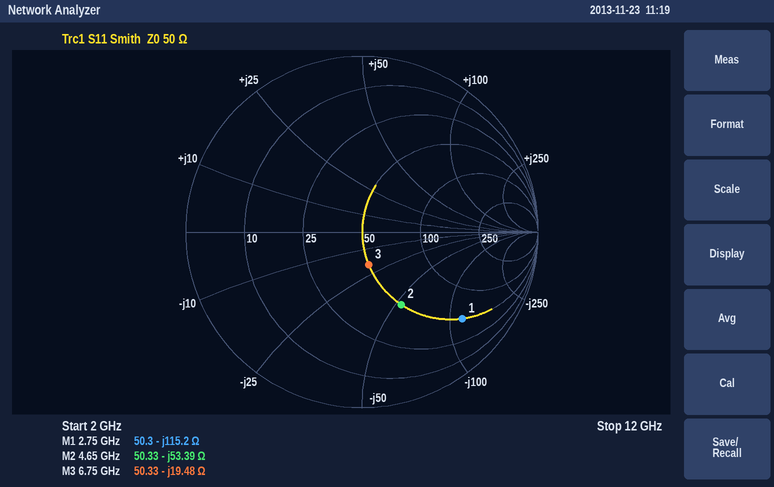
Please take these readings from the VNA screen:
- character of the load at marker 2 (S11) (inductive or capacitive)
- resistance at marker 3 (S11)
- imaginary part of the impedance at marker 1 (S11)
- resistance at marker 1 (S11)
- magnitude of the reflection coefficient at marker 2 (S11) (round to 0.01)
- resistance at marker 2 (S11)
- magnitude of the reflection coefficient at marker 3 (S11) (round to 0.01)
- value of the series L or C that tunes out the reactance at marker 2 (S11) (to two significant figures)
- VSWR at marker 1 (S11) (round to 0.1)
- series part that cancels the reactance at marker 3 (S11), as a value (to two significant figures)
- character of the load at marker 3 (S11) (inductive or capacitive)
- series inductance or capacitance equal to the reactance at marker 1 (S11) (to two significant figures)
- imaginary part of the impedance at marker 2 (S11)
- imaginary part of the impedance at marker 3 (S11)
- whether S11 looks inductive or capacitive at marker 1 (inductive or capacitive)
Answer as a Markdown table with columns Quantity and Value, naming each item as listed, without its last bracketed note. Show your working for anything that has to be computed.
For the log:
| Quantity | Value |
|---|---|
| character of the load at marker 2 (S11) | capacitive |
| resistance at marker 3 | 50.33 Ω |
| imaginary part of the impedance at marker 1 | -115.2 Ω |
| resistance at marker 1 | 50.3 Ω |
| magnitude of the reflection coefficient at marker 2 (S11) | 0.47 |
| resistance at marker 2 | 50.33 Ω |
| magnitude of the reflection coefficient at marker 3 (S11) | 0.19 |
| value of the series L or C that tunes out the reactance at marker 2 (S11) | L = 53.39 Ω/(2π × 4.65 GHz) ≈ 1.8 nH |
| VSWR at marker 1 (S11) | 7.1 |
| series part that cancels the reactance at marker 3 (S11), as a value | L = 19.48 Ω/(2π × 6.75 GHz) ≈ 459 pH, so 460 pH to two significant figures |
| character of the load at marker 3 (S11) | capacitive |
| series inductance or capacitance equal to the reactance at marker 1 (S11) | C = 1/(2π × 2.75 GHz × 115.2 Ω) ≈ 502 fF, so 500 fF to two significant figures |
| imaginary part of the impedance at marker 2 | -53.39 Ω |
| imaginary part of the impedance at marker 3 | -19.48 Ω |
| whether S11 looks inductive or capacitive at marker 1 | capacitive |
